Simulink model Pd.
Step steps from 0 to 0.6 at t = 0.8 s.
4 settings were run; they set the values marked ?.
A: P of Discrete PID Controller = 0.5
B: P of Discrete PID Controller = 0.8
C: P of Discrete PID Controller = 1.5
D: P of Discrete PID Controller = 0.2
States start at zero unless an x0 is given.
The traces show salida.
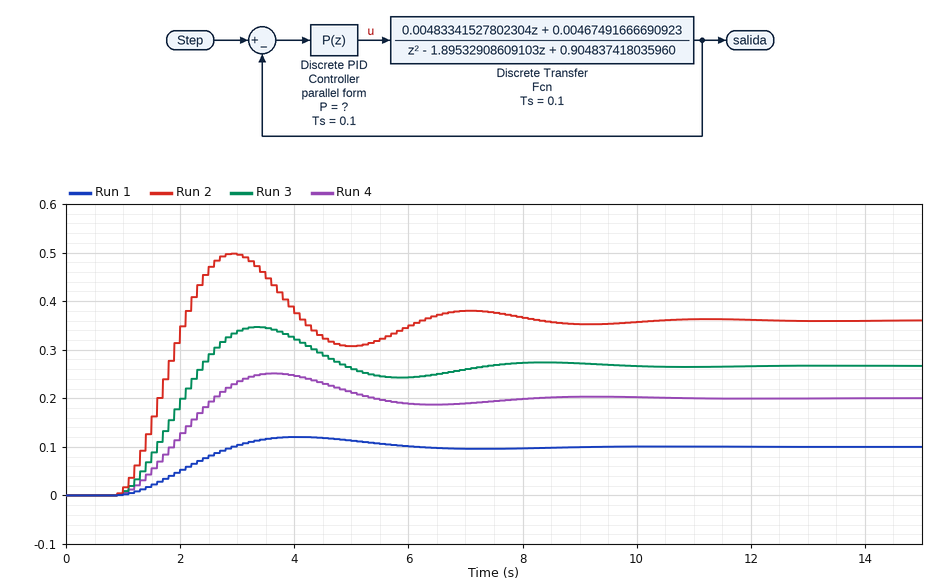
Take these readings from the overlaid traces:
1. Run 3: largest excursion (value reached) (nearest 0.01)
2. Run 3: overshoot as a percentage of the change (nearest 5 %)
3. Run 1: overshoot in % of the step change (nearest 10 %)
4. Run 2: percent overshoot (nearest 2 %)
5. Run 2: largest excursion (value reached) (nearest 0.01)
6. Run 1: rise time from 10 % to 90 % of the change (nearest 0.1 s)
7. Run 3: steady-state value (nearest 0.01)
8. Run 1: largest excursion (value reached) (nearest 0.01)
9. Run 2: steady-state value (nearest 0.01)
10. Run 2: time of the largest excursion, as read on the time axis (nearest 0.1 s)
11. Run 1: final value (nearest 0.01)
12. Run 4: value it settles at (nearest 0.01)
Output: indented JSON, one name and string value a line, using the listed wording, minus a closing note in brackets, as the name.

{
  "Run 3: largest excursion (value reached)": "0.35",
  "Run 3: overshoot as a percentage of the change": "30 %",
  "Run 1: overshoot in % of the step change": "20 %",
  "Run 2: percent overshoot": "38 %",
  "Run 2: largest excursion (value reached)": "0.50",
  "Run 1: rise time from 10 % to 90 % of the change": "1.4 s",
  "Run 3: steady-state value": "0.27",
  "Run 1: largest excursion (value reached)": "0.12",
  "Run 2: steady-state value": "0.36",
  "Run 2: time of the largest excursion, as read on the time axis": "2.9 s",
  "Run 1: final value": "0.10",
  "Run 4: value it settles at": "0.20"
}
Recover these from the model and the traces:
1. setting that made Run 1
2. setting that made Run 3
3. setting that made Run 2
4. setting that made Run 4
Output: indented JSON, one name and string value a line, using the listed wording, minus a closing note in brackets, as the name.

{
  "setting that made Run 1": "D",
  "setting that made Run 3": "B",
  "setting that made Run 2": "C",
  "setting that made Run 4": "A"
}
